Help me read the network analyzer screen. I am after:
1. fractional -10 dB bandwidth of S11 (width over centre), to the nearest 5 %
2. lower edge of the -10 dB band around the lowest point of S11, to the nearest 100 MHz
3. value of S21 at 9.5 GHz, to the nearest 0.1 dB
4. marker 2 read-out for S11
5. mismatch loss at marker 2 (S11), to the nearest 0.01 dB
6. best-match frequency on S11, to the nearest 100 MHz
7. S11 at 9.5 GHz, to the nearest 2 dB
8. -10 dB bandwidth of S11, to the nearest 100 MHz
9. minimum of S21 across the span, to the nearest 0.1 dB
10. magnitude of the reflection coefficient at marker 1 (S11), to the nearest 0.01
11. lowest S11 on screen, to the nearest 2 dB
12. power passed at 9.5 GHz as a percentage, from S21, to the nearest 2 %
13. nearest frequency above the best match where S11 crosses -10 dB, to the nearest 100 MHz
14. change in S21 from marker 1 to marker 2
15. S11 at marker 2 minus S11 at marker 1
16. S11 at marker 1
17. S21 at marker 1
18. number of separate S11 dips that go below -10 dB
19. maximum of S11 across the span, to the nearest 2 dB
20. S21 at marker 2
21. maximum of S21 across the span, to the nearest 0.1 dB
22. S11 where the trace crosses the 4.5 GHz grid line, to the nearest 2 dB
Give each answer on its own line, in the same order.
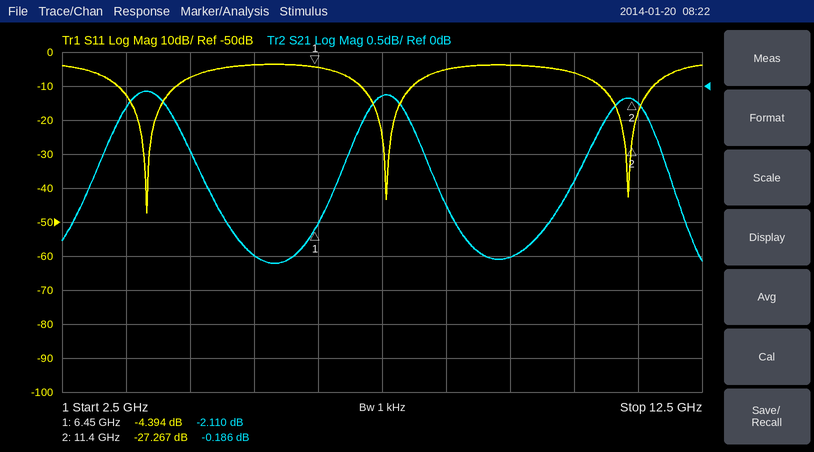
25 %
3.4 GHz
-2.5 dB
-27.267 dB
0.01 dB
3.8 GHz
-4 dB
900 MHz
-2.6 dB
0.60
-48 dB
56 %
4.3 GHz
1.924 dB
-22.873 dB
-4.394 dB
-2.110 dB
3
-4 dB
-0.186 dB
-0.1 dB
-8 dB
